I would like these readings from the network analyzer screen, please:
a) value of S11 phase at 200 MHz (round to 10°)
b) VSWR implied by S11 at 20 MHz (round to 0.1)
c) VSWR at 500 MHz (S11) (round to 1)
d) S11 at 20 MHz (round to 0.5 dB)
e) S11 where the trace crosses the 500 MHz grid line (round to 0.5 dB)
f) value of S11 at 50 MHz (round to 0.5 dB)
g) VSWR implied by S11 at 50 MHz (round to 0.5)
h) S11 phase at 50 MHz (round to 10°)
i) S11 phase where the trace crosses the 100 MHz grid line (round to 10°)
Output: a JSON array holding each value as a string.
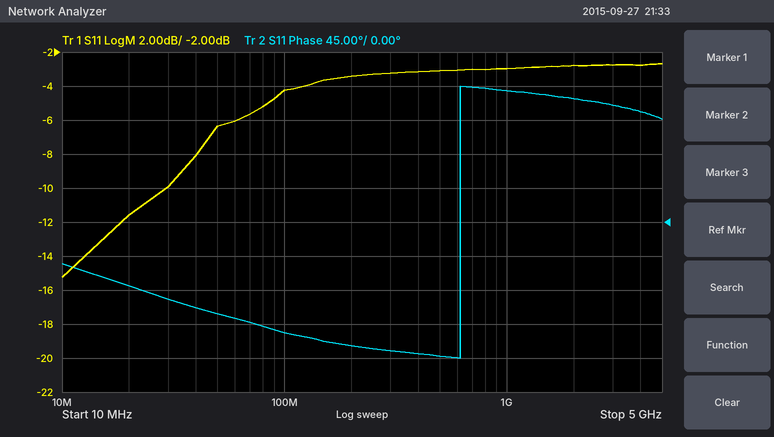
["-160°", "1.7", "6", "-11.5 dB", "-3.0 dB", "-6.5 dB", "3.0", "-120°", "-150°"]
